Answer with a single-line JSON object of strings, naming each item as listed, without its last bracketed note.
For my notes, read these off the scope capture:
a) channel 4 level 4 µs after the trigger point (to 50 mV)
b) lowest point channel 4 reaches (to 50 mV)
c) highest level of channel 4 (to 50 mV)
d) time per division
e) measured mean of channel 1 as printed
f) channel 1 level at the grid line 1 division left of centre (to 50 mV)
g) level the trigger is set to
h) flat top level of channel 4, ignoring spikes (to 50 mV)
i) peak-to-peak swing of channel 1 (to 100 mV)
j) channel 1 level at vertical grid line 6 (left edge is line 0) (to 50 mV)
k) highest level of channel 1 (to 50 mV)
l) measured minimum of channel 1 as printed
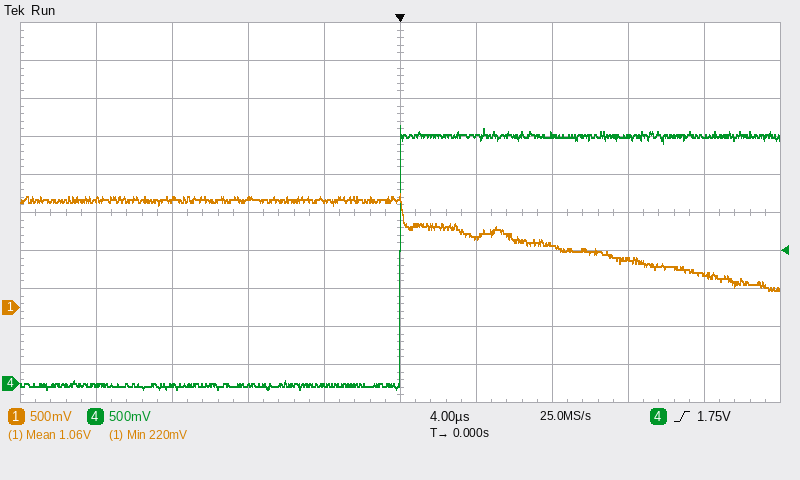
{"channel 4 level 4 µs after the trigger point": "3.25 V", "lowest point channel 4 reaches": "-100 mV", "highest level of channel 4": "3.40 V", "time per division": "4 µs", "measured mean of channel 1 as printed": "1.06 V", "channel 1 level at the grid line 1 division left of centre": "1.40 V", "level the trigger is set to": "1.75 V", "flat top level of channel 4, ignoring spikes": "3.25 V", "peak-to-peak swing of channel 1": "1.30 V", "channel 1 level at vertical grid line 6 (left edge is line 0)": "950 mV", "highest level of channel 1": "1.50 V", "measured minimum of channel 1 as printed": "220 mV"}
